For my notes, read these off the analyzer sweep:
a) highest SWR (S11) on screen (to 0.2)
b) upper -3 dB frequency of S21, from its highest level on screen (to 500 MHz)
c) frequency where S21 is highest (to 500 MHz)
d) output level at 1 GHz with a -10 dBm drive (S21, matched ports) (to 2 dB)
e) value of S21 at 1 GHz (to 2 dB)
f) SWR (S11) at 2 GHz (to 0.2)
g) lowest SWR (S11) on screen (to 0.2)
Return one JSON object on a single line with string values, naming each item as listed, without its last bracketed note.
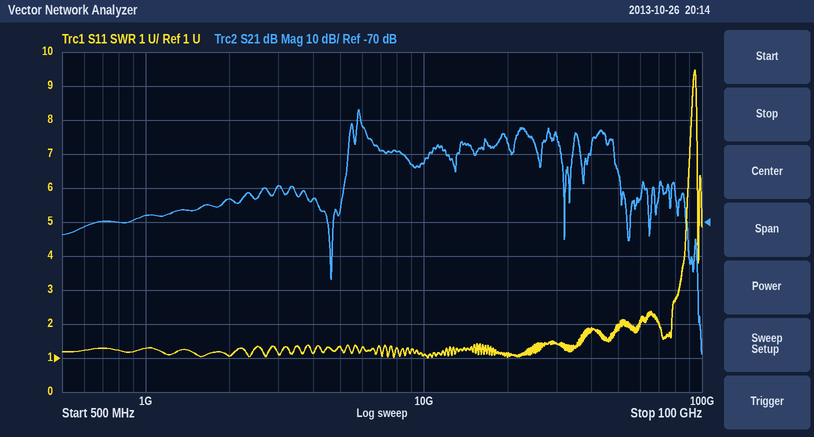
{"highest SWR (S11) on screen": "9.4", "upper -3 dB frequency of S21, from its highest level on screen": "6.0 GHz", "frequency where S21 is highest": "6.0 GHz", "output level at 1 GHz with a -10 dBm drive (S21, matched ports)": "-78 dBm", "value of S21 at 1 GHz": "-68 dB", "SWR (S11) at 2 GHz": "1.0", "lowest SWR (S11) on screen": "1.0"}
